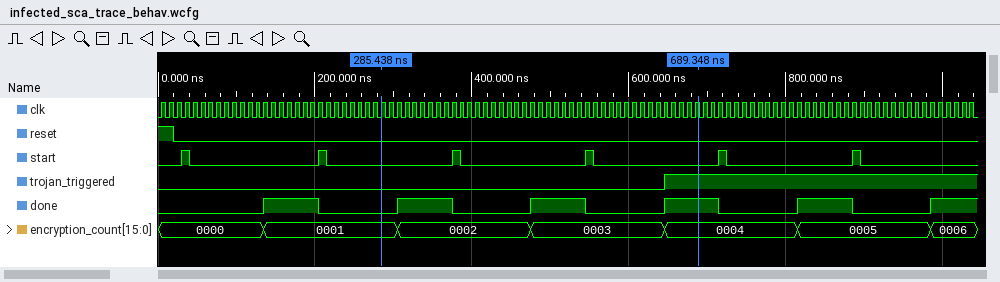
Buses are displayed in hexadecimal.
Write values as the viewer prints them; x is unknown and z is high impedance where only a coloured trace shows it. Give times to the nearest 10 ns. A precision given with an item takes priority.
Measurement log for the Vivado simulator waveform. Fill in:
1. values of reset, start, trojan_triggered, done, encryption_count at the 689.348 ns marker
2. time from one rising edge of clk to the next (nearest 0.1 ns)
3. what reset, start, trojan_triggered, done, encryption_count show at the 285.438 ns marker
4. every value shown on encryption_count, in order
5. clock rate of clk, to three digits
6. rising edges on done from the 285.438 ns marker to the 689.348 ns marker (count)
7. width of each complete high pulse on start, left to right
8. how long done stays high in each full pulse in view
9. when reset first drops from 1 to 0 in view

reset=0, start=0, trojan_triggered=1, done=1, encryption_count=0004
10 ns
reset=0, start=0, trojan_triggered=0, done=0, encryption_count=0001
0000, 0001, 0002, 0003, 0004, 0005, 0006
100 MHz
3
10 ns, 10 ns, 10 ns, 10 ns, 10 ns, 10 ns
70 ns, 70 ns, 70 ns, 70 ns, 70 ns
20 ns
